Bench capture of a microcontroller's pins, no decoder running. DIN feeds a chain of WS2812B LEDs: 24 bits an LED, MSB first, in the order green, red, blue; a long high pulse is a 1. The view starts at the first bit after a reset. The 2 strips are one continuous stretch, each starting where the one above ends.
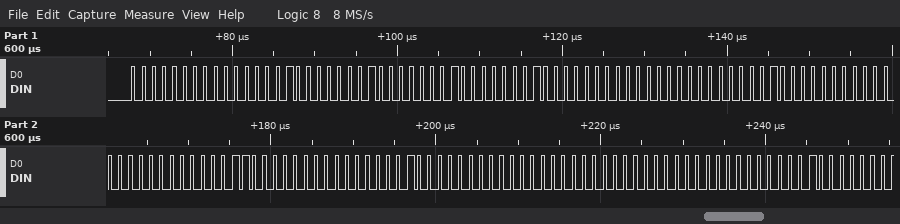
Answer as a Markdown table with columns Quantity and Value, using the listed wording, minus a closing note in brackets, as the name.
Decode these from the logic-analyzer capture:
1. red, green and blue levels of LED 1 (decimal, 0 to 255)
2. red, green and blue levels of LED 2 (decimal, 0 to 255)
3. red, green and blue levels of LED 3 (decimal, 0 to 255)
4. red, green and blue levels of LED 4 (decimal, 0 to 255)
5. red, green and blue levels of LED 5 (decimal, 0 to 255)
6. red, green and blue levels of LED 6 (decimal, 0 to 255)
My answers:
| Quantity | Value |
|---|---|
| red, green and blue levels of LED 1 | 1, 0, 1 |
| red, green and blue levels of LED 2 | 1, 1, 0 |
| red, green and blue levels of LED 3 | 2, 0, 0 |
| red, green and blue levels of LED 4 | 3, 0, 0 |
| red, green and blue levels of LED 5 | 0, 1, 0 |
| red, green and blue levels of LED 6 | 0, 0, 2 |
